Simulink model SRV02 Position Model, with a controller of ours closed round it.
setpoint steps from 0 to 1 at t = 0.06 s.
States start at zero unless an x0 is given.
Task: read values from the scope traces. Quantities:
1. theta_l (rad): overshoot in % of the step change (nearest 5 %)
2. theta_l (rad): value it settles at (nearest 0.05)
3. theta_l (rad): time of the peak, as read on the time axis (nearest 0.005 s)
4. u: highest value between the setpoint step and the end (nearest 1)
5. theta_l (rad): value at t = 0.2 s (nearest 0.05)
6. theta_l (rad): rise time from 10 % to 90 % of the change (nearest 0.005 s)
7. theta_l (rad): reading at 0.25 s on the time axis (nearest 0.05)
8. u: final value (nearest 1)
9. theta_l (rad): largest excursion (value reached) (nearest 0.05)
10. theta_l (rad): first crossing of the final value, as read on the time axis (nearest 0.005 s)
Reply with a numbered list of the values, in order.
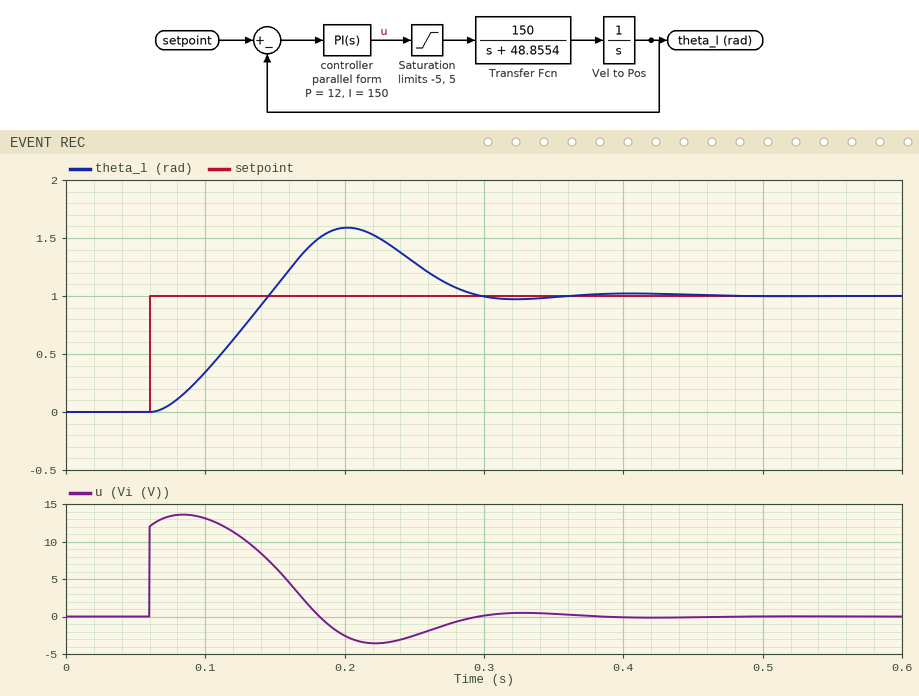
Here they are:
1. 60 %
2. 1.00
3. 0.200 s
4. 14
5. 1.60
6. 0.060 s
7. 1.30
8. 0
9. 1.60
10. 0.145 s
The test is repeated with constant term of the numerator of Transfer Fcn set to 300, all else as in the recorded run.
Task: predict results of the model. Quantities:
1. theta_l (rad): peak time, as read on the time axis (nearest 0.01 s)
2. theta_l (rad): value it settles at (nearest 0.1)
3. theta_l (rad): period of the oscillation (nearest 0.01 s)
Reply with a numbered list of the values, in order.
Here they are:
1. 0.14 s
2. 1.0
3. 0.12 s
